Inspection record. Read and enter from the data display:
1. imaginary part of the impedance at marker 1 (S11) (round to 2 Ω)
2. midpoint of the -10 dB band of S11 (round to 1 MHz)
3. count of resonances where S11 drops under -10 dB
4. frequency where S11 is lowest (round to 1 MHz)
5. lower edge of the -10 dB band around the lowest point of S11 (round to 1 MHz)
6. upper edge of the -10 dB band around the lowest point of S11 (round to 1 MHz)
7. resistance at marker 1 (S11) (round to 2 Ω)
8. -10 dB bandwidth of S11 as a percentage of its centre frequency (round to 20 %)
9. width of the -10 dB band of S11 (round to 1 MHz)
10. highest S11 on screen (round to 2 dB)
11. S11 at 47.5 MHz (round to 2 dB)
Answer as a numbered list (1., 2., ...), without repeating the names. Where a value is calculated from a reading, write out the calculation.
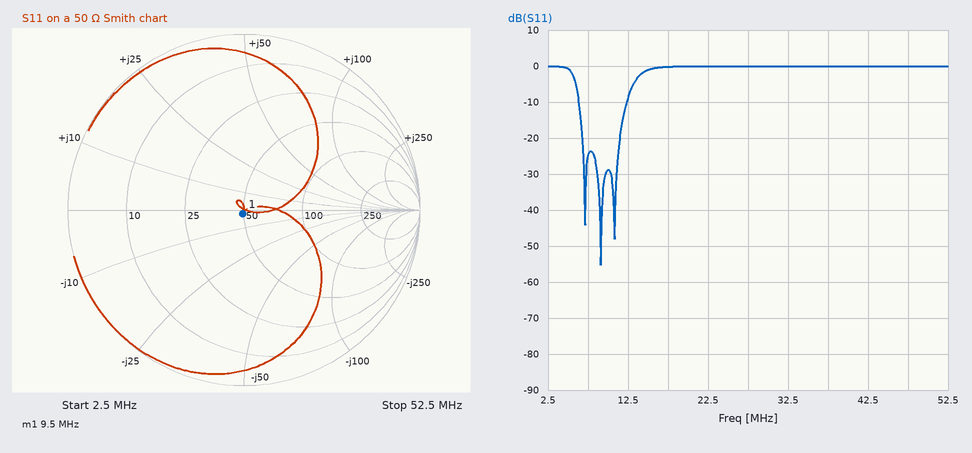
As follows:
1. -2 Ω
2. 9 MHz
3. 3
4. 9 MHz
5. 6 MHz
6. 12 MHz
7. 50 Ω
8. 6 MHz / 9 MHz ≈ 66.7 %, so 60 % to the nearest 20 %
9. 12 MHz − 6 MHz = 6 MHz
10. 0 dB
11. 0 dB
